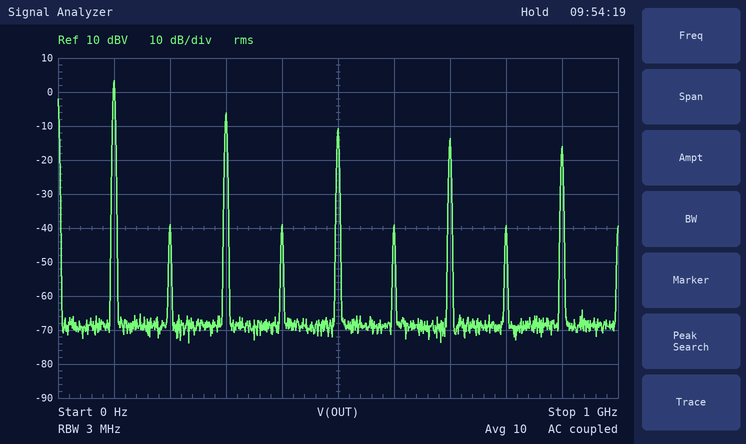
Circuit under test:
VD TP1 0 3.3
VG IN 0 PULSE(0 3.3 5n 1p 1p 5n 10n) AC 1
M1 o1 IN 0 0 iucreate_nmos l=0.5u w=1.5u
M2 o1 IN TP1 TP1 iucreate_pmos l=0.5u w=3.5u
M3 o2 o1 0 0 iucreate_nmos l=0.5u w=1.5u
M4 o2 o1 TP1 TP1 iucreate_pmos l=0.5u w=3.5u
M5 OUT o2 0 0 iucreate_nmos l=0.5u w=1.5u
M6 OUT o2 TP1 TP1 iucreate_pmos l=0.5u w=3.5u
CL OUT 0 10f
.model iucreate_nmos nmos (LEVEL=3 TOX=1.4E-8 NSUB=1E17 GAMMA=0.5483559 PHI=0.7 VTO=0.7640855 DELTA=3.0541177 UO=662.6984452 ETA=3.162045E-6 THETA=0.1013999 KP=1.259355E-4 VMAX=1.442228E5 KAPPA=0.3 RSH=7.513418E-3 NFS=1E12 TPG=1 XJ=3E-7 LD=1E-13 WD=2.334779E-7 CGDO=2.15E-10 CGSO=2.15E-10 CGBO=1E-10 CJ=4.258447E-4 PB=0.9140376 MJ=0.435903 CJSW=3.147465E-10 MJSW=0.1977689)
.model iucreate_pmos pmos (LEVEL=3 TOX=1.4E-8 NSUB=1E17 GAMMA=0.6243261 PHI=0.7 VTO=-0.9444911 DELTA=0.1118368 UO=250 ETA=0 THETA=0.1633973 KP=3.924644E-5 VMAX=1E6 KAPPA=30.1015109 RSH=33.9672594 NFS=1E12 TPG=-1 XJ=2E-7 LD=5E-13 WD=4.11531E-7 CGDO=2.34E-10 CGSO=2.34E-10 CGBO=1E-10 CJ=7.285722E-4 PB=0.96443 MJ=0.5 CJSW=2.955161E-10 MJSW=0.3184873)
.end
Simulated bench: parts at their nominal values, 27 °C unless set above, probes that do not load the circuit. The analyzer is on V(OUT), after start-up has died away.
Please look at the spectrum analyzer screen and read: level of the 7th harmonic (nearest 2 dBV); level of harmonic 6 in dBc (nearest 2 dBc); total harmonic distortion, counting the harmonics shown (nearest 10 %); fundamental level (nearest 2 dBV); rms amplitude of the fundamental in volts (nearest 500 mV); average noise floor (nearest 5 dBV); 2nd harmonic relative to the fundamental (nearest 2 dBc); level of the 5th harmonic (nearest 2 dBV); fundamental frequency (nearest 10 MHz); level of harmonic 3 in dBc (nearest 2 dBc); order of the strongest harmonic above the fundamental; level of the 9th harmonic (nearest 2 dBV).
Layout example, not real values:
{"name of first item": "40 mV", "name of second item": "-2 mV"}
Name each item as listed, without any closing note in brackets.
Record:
{"level of the 7th harmonic": "-14 dBV", "level of harmonic 6 in dBc": "-42 dBc", "total harmonic distortion, counting the harmonics shown": "40 %", "fundamental level": "4 dBV", "rms amplitude of the fundamental in volts": "1.5 V", "average noise floor": "-70 dBV", "2nd harmonic relative to the fundamental": "-42 dBc", "level of the 5th harmonic": "-10 dBV", "fundamental frequency": "100 MHz", "level of harmonic 3 in dBc": "-10 dBc", "order of the strongest harmonic above the fundamental": "3", "level of the 9th harmonic": "-16 dBV"}
